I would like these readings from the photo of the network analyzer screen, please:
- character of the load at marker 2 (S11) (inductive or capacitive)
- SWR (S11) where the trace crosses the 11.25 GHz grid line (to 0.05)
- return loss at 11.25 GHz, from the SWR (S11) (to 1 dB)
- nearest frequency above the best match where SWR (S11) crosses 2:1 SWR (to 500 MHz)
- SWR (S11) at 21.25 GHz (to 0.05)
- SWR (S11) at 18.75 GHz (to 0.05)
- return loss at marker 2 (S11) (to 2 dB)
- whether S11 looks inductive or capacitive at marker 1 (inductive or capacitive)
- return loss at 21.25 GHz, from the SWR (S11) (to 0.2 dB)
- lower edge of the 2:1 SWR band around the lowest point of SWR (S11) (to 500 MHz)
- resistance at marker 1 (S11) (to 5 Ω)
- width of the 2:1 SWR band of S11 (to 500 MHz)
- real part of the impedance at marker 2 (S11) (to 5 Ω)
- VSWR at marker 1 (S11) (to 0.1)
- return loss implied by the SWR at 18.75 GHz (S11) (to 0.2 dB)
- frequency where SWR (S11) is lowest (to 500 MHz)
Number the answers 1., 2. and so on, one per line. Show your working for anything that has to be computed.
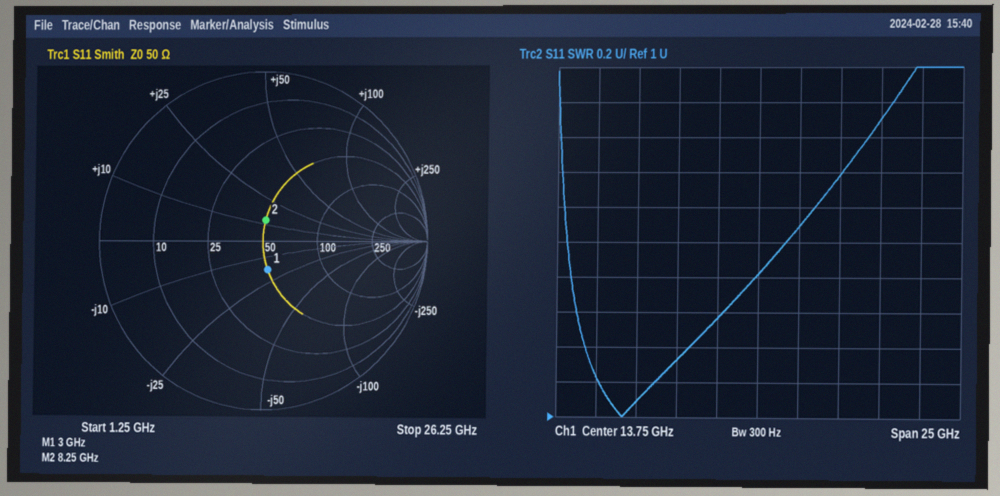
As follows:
1. inductive
2. 1.55
3. −20 log10((1.55 − 1)/(1.55 + 1)) ≈ 13 dB
4. 15.5 GHz
5. 2.70
6. 2.40
7. 18 dB
8. capacitive
9. −20 log10((2.7 − 1)/(2.7 + 1)) ≈ 6.8 dB
10. 2.0 GHz
11. 50 Ω
12. 15.5 GHz − 2.0 GHz = 13.5 GHz
13. 50 Ω
14. 1.4
15. −20 log10((2.4 − 1)/(2.4 + 1)) ≈ 7.71 dB, so 7.8 dB to the nearest 0.2 dB
16. 5.5 GHz
